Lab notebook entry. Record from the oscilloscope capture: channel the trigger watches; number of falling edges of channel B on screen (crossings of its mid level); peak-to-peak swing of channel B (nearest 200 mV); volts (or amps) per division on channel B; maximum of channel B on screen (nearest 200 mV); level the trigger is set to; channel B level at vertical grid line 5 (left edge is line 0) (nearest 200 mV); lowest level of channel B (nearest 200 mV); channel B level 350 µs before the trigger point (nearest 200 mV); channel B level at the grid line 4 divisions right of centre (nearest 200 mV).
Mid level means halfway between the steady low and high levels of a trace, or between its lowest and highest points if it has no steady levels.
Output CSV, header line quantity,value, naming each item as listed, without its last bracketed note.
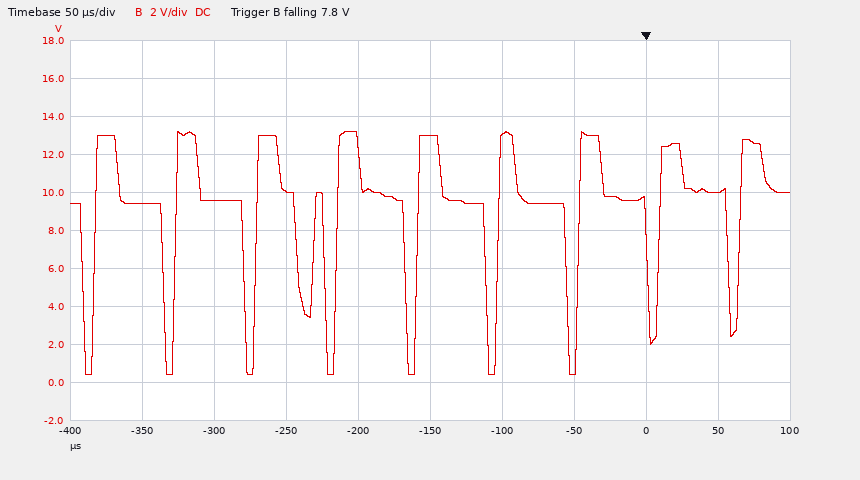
quantity,value
channel the trigger watches,channel B
number of falling edges of channel B on screen,10
peak-to-peak swing of channel B,12.8 V
volts (or amps) per division on channel B,2 V
maximum of channel B on screen,13.2 V
level the trigger is set to,7.8 V
channel B level at vertical grid line 5 (left edge is line 0),13.0 V
lowest level of channel B,400 mV
channel B level 350 µs before the trigger point,9.4 V
channel B level at the grid line 4 divisions right of centre,10.0 V
